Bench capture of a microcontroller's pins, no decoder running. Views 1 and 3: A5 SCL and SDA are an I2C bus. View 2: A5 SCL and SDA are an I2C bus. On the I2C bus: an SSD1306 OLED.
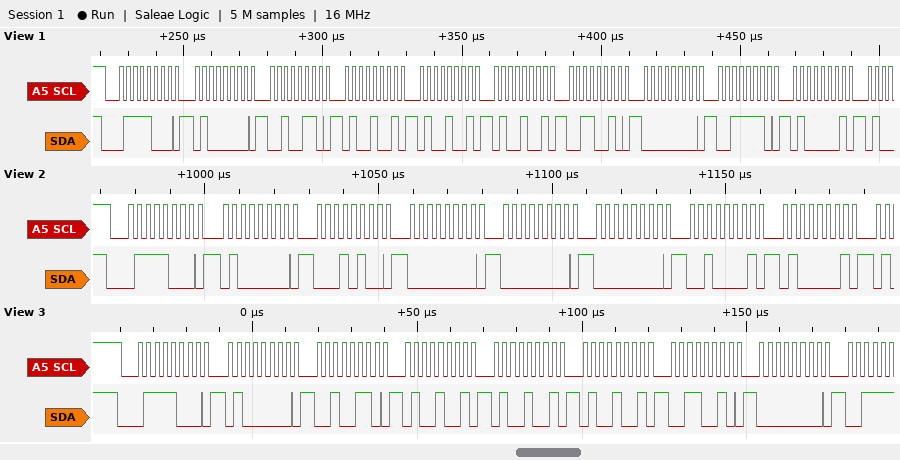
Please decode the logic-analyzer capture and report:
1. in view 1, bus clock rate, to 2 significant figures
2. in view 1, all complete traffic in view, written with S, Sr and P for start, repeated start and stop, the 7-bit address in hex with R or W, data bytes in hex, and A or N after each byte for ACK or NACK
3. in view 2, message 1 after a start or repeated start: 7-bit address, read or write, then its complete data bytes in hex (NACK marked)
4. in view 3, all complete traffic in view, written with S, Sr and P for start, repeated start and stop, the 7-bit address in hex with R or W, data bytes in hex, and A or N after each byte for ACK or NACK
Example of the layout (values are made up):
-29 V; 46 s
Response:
400 kHz; S 3CW A 40 A 26 A 49 A 49 A 49 A 32 A 00 A 3E A 41 A; 0x3C write: 40 14 00 00 00 21 41; S 3CW A 40 A 26 A 49 A 49 A 49 A 32 A 00 A
